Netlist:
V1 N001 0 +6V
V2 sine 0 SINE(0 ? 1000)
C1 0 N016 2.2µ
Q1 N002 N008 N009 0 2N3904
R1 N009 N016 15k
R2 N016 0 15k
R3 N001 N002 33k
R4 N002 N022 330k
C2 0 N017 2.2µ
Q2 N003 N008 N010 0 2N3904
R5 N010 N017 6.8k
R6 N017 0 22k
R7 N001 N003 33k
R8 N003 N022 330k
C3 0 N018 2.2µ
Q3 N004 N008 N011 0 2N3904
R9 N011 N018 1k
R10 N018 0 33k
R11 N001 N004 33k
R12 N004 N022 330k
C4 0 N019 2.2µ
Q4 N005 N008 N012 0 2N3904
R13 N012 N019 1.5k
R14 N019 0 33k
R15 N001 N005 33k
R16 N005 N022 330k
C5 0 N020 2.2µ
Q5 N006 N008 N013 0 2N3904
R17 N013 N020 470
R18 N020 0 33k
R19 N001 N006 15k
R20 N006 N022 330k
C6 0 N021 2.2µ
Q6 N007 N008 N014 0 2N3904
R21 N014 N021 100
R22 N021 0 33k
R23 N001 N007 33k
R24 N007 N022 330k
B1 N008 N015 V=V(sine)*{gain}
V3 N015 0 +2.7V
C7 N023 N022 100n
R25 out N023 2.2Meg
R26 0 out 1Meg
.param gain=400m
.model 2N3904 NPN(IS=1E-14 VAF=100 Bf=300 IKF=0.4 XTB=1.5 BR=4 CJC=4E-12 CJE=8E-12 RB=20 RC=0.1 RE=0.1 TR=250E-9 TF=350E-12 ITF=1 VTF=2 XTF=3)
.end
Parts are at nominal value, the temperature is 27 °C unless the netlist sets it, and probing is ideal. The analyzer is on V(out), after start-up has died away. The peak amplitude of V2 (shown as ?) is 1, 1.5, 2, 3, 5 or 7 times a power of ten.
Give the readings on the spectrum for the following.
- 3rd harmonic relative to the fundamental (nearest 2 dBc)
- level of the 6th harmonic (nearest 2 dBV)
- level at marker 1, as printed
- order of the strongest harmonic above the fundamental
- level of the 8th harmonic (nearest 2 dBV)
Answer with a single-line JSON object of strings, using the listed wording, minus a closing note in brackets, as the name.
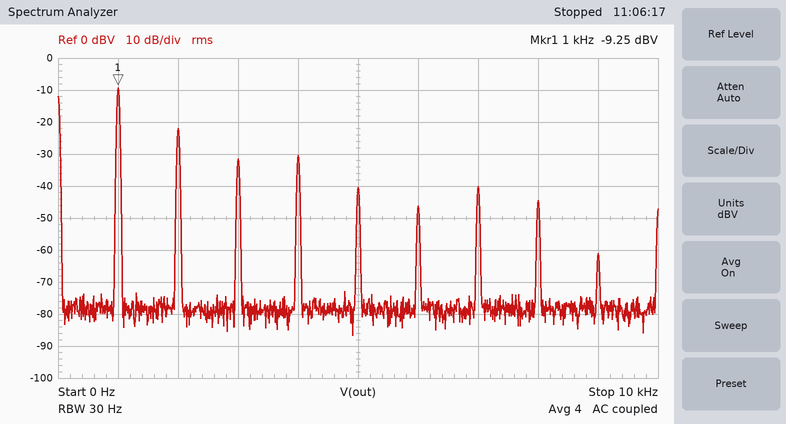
{"3rd harmonic relative to the fundamental": "-22 dBc", "level of the 6th harmonic": "-46 dBV", "level at marker 1, as printed": "-9.25 dBV", "order of the strongest harmonic above the fundamental": "2", "level of the 8th harmonic": "-44 dBV"}
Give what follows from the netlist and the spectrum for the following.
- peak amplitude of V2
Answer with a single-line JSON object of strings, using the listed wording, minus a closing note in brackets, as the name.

{"peak amplitude of V2": "500 mV"}
